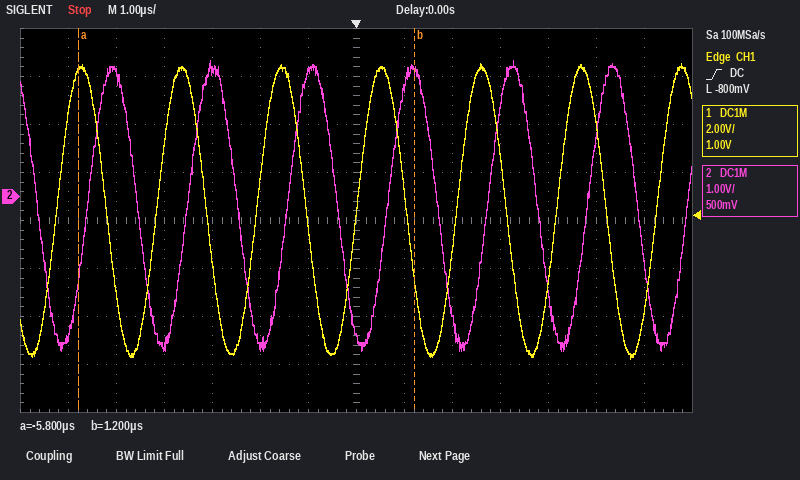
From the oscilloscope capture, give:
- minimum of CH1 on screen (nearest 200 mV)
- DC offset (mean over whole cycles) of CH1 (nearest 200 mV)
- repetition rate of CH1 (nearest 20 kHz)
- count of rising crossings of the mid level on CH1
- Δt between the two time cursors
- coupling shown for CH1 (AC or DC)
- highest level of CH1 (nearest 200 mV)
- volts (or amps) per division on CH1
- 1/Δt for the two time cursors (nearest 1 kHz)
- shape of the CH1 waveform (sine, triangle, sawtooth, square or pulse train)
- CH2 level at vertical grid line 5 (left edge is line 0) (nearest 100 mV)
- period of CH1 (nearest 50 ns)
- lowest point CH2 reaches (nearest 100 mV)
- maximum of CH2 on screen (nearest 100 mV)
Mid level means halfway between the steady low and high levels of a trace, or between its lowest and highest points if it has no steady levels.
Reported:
-6.8 V
-600 mV
480 kHz
7
7.0 µs
DC
5.6 V
2 V
143 kHz
sine
-3.1 V
2.10 µs
-3.2 V
2.8 V
